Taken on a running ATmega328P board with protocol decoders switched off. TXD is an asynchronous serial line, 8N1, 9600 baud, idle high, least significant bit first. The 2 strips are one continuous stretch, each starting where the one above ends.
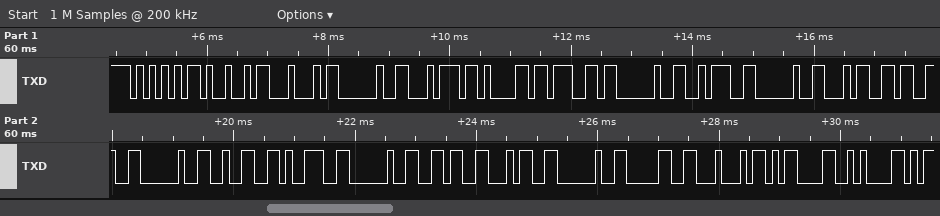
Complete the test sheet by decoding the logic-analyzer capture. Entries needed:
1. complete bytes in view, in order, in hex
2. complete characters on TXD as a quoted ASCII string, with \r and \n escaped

55 49 44 20 74 61 67 20 3A 20 34 33 20 32 39 20 36 34 20 30 44 0D 0A
"UID tag : 43 29 64 0D\r\n"
